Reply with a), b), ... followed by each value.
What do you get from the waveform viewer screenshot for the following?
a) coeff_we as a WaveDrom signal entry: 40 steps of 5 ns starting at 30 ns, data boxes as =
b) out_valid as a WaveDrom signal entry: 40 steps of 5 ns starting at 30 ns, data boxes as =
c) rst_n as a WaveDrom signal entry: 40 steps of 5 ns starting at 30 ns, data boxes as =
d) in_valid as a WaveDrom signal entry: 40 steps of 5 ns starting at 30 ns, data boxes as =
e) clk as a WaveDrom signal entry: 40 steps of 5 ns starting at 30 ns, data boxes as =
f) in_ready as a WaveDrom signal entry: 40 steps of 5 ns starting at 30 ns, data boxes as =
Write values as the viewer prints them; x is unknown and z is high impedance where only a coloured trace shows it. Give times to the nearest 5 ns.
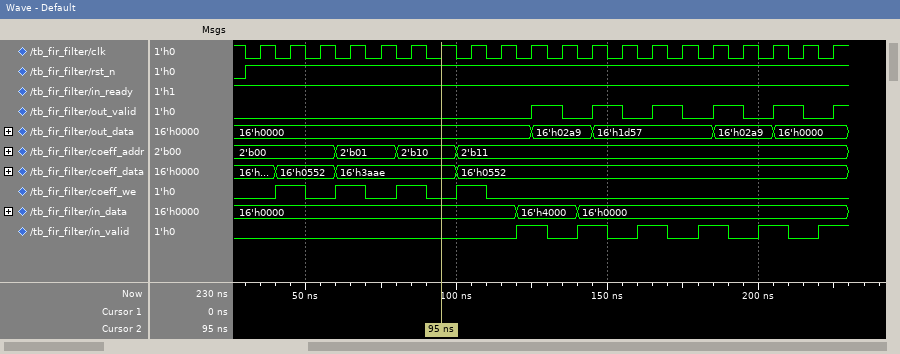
a) {name: 'coeff_we', wave: '0.1.0.1.0.1.0.1.0.......................'}
b) {name: 'out_valid', wave: '0..................1.0.1.0.1.0.1.0.1.0.1'}
c) {name: 'rst_n', wave: '1.......................................'}
d) {name: 'in_valid', wave: '0.................1.0.1.0.1.0.1.0.1.0.1.'}
e) {name: 'clk', wave: '0101010101010101010101010101010101010101'}
f) {name: 'in_ready', wave: '1.......................................'}
